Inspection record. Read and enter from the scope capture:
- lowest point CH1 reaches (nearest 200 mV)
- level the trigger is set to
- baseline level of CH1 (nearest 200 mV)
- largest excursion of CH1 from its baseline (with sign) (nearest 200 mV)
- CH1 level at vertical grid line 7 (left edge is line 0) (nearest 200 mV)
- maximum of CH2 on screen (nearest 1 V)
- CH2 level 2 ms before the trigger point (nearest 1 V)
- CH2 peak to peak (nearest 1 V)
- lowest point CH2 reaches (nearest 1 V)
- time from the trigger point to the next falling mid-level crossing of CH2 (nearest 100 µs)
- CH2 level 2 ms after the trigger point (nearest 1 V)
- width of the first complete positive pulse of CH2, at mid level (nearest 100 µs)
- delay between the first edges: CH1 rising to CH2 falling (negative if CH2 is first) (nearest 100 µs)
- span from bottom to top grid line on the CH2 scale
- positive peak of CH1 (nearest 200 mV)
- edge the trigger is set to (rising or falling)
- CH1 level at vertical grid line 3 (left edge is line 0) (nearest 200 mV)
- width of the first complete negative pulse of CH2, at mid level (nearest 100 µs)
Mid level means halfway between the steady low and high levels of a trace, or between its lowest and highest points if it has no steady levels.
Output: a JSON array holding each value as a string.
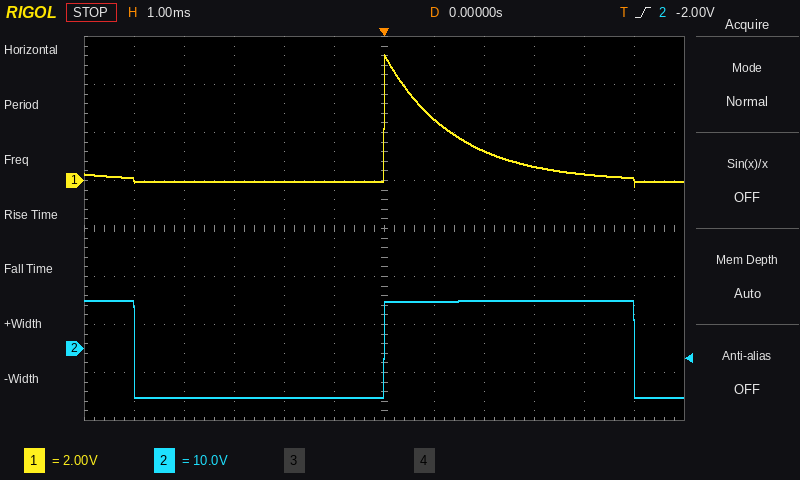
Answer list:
["-200 mV", "-2.00 V", "0.0 V", "+5.2 V", "2.6 V", "10 V", "-10 V", "20 V", "-10 V", "5.0 ms", "10 V", "5.0 ms", "-5.0 ms", "80 V", "5.2 V", "rising", "0.0 V", "5.0 ms"]
